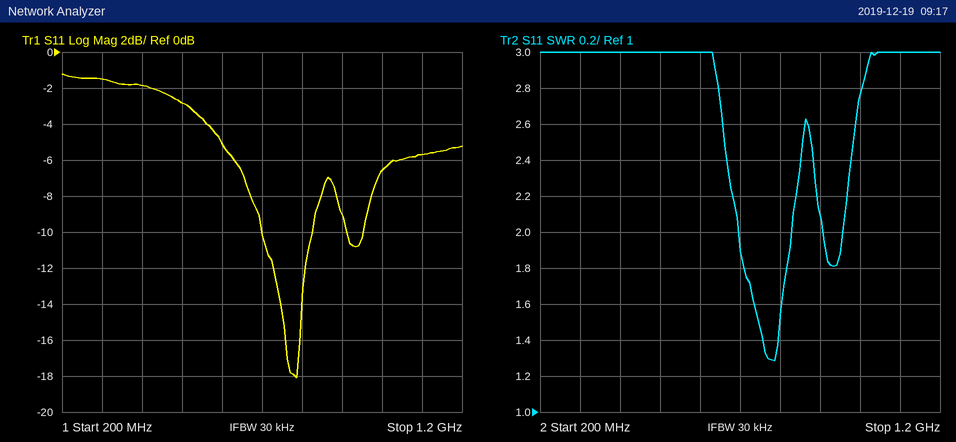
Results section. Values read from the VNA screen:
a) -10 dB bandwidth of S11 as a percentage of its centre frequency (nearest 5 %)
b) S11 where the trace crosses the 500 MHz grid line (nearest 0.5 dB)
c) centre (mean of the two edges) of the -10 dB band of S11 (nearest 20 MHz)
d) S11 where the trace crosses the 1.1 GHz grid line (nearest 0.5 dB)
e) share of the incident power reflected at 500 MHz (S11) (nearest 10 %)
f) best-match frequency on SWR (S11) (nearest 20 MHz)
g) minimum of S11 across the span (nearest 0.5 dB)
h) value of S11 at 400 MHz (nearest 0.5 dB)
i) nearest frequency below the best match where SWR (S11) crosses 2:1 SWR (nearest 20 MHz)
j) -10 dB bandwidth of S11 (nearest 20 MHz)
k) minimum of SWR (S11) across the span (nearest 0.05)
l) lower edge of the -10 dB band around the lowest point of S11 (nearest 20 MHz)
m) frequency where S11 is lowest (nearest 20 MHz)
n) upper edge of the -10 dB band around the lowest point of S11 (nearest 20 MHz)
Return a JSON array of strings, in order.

["15 %", "-3.0 dB", "760 MHz", "-5.5 dB", "50 %", "780 MHz", "-18.0 dB", "-2.0 dB", "700 MHz", "120 MHz", "1.30", "700 MHz", "780 MHz", "820 MHz"]
